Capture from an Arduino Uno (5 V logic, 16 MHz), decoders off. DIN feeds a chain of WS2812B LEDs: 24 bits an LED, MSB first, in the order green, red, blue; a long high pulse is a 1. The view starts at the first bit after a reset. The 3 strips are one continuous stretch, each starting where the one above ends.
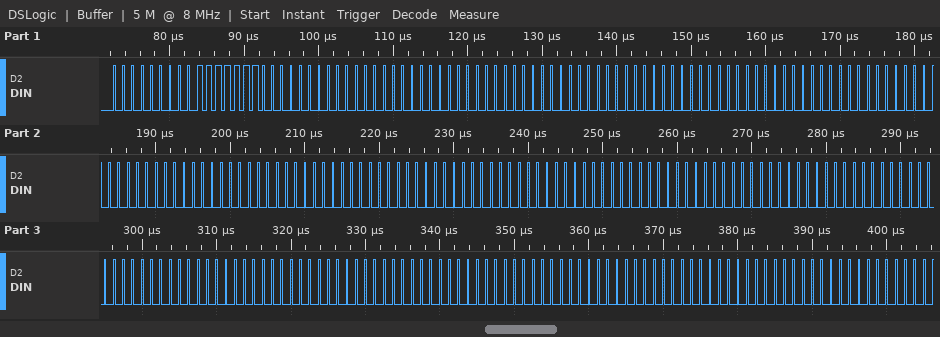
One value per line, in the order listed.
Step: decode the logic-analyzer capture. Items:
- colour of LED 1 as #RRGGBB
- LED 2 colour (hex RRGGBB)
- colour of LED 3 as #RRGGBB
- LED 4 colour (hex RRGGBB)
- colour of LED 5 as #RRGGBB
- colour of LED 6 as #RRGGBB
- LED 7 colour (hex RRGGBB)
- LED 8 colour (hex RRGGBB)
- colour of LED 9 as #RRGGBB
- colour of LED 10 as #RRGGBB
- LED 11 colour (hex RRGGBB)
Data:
#7F0000
#000000
#000000
#000000
#000000
#000000
#000000
#000000
#000000
#000000
#000000
